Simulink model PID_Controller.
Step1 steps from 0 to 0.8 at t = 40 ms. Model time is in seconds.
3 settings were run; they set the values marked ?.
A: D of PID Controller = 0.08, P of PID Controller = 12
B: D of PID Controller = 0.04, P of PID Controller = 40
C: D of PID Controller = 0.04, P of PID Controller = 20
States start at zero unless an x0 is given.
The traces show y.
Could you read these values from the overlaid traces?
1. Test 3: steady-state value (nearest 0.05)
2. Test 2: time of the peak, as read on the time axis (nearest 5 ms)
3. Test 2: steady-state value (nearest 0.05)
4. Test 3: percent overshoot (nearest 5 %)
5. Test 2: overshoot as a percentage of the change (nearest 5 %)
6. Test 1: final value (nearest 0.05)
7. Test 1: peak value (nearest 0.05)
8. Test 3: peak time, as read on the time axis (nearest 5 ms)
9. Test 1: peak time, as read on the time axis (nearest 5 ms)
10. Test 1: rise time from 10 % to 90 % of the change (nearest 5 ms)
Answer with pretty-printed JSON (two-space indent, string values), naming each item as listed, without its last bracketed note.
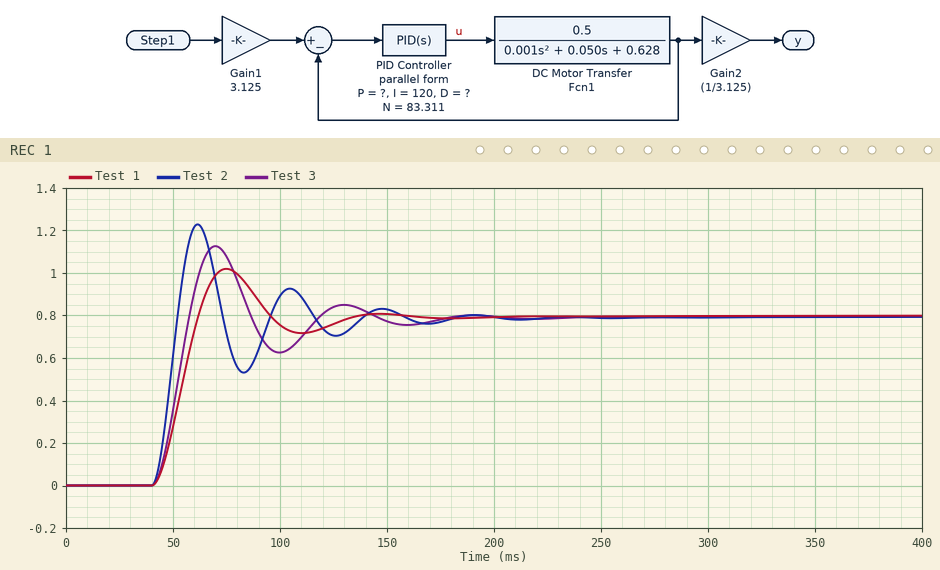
{
  "Test 3: steady-state value": "0.80",
  "Test 2: time of the peak, as read on the time axis": "60 ms",
  "Test 2: steady-state value": "0.80",
  "Test 3: percent overshoot": "40 %",
  "Test 2: overshoot as a percentage of the change": "55 %",
  "Test 1: final value": "0.80",
  "Test 1: peak value": "1.00",
  "Test 3: peak time, as read on the time axis": "70 ms",
  "Test 1: peak time, as read on the time axis": "75 ms",
  "Test 1: rise time from 10 % to 90 % of the change": "15 ms"
}
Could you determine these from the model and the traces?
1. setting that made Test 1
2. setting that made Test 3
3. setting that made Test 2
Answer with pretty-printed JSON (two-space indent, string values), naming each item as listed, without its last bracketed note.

{
  "setting that made Test 1": "A",
  "setting that made Test 3": "C",
  "setting that made Test 2": "B"
}
